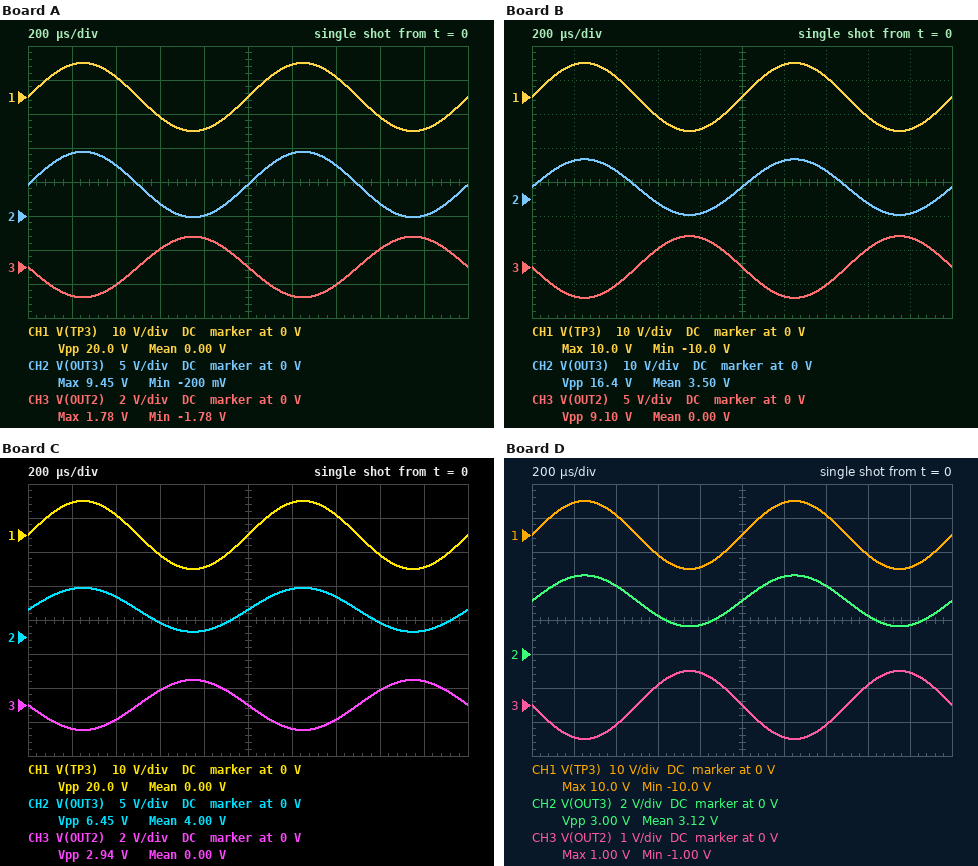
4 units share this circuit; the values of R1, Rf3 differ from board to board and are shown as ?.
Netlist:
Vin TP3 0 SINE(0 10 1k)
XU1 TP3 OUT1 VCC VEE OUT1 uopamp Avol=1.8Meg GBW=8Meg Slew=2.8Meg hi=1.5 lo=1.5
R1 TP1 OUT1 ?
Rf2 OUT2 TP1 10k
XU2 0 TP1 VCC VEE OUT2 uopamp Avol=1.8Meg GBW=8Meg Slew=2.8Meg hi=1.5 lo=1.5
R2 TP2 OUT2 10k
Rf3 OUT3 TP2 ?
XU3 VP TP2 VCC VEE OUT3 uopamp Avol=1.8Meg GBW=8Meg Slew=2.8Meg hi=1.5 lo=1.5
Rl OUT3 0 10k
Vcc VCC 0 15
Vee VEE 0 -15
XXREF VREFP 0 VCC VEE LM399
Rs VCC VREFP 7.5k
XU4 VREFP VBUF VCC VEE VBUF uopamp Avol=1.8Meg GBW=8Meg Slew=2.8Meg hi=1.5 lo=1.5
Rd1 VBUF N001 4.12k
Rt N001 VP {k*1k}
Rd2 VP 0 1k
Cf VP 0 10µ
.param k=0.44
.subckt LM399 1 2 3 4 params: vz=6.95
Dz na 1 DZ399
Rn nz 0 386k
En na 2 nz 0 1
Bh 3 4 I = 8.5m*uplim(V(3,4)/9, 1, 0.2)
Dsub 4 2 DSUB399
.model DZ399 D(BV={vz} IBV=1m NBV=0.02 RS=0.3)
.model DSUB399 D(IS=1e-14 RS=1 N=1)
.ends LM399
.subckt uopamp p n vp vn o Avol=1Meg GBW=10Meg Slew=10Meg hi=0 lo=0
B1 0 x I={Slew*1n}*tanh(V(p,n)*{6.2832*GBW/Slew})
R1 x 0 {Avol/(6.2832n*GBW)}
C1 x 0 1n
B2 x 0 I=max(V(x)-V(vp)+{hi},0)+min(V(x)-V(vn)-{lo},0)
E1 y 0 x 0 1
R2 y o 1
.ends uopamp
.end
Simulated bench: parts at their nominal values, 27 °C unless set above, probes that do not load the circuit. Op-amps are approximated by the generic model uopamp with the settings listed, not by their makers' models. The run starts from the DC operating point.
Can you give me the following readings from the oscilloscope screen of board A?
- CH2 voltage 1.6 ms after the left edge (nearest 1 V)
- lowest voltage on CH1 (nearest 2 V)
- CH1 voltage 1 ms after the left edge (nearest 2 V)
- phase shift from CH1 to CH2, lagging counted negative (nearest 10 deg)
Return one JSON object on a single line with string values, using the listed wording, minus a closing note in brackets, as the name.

{"CH2 voltage 1.6 ms after the left edge": "2 V", "lowest voltage on CH1": "-10 V", "CH1 voltage 1 ms after the left edge": "0 V", "phase shift from CH1 to CH2, lagging counted negative": "0 deg"}
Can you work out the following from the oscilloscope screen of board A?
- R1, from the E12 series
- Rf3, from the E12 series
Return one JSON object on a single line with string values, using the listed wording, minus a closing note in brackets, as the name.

{"R1, from the E12 series": "56 kΩ", "Rf3, from the E12 series": "27 kΩ"}
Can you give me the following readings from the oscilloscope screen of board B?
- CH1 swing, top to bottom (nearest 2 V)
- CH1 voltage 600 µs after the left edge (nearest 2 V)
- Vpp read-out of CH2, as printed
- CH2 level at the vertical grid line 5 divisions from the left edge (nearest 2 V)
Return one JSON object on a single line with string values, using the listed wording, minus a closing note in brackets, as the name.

{"CH1 swing, top to bottom": "20 V", "CH1 voltage 600 µs after the left edge": "-6 V", "Vpp read-out of CH2, as printed": "16.4 V", "CH2 level at the vertical grid line 5 divisions from the left edge": "4 V"}
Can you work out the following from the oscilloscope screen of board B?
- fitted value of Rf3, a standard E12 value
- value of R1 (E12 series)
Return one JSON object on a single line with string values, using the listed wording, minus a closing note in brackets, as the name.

{"fitted value of Rf3, a standard E12 value": "18 kΩ", "value of R1": "22 kΩ"}
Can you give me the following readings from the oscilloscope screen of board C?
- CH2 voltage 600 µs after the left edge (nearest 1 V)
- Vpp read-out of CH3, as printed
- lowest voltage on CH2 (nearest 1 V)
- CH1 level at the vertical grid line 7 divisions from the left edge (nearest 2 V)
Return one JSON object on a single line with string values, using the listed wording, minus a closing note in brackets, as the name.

{"CH2 voltage 600 µs after the left edge": "2 V", "Vpp read-out of CH3, as printed": "2.94 V", "lowest voltage on CH2": "1 V", "CH1 level at the vertical grid line 7 divisions from the left edge": "6 V"}
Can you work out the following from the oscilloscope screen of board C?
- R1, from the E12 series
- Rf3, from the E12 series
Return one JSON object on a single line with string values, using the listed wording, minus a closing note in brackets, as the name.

{"R1, from the E12 series": "68 kΩ", "Rf3, from the E12 series": "22 kΩ"}
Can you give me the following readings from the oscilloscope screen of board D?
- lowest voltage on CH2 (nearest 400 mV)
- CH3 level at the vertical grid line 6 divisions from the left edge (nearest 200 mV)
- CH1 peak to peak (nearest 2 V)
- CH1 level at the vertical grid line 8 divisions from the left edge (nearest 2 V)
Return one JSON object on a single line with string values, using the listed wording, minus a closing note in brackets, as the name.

{"lowest voltage on CH2": "1.6 V", "CH3 level at the vertical grid line 6 divisions from the left edge": "-1.0 V", "CH1 peak to peak": "20 V", "CH1 level at the vertical grid line 8 divisions from the left edge": "-6 V"}
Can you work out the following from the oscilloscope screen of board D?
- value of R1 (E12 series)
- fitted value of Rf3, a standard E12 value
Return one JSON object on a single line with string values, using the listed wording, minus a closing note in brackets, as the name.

{"value of R1": "100 kΩ", "fitted value of Rf3, a standard E12 value": "15 kΩ"}
